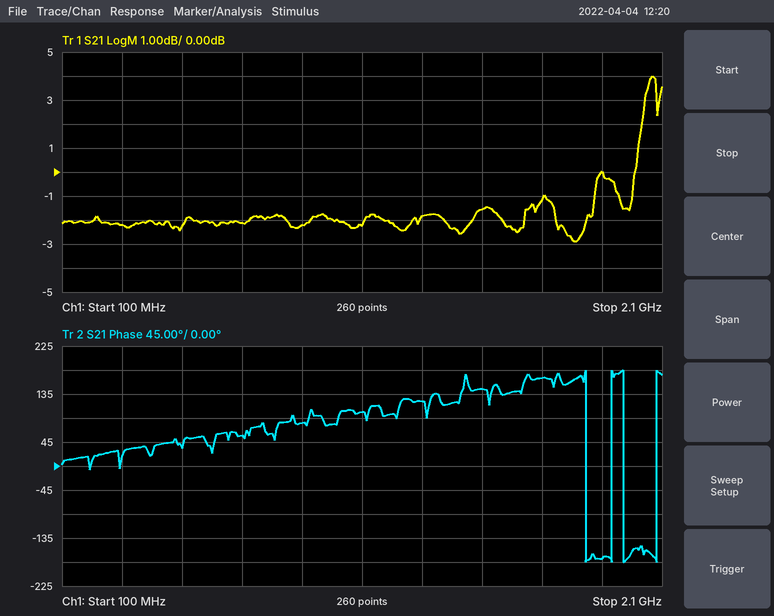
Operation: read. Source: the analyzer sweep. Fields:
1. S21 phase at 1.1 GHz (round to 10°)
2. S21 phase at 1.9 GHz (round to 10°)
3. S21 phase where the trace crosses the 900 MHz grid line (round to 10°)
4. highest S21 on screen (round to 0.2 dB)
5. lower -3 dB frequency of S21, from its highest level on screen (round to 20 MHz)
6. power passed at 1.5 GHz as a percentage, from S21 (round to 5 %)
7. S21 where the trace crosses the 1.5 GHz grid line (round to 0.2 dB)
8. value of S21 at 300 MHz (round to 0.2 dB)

100°
-170°
80°
4.0 dB
2.02 GHz
70 %
-1.6 dB
-2.2 dB
